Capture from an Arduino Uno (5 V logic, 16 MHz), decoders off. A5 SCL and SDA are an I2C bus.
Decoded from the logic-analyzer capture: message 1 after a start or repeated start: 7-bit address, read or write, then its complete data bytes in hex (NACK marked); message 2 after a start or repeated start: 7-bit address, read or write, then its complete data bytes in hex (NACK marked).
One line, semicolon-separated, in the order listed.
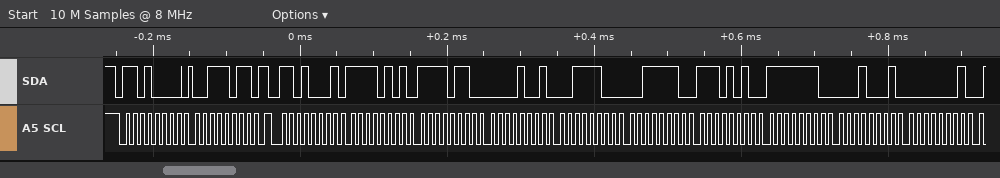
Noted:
0x68 write: 3B; 0x68 read: F5 F6 09 3C 3E EA FE 11 01
